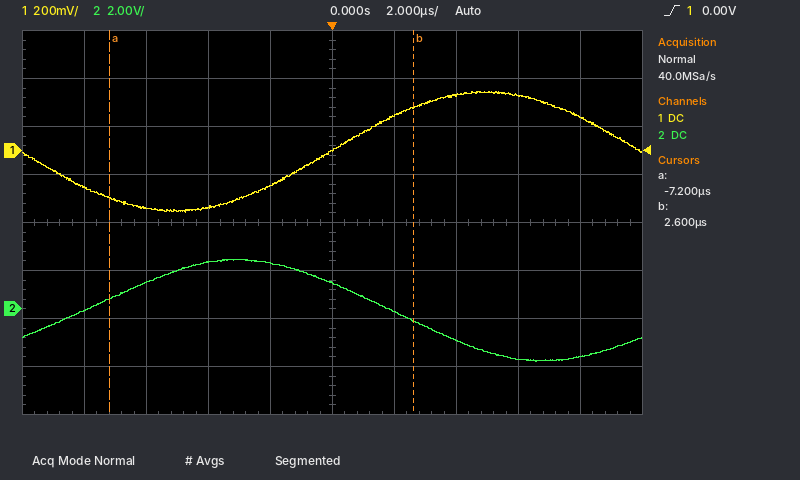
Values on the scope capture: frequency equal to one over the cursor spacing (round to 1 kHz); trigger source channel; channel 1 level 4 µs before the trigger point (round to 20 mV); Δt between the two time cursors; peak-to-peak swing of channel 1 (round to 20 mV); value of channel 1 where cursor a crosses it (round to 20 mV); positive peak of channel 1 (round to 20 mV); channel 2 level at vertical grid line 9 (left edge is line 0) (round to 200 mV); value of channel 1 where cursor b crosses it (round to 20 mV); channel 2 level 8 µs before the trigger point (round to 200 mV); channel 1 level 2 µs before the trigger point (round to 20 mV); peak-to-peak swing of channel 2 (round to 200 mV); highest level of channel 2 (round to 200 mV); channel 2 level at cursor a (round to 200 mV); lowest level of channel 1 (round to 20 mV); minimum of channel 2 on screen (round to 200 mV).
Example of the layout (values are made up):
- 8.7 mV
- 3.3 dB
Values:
- 102 kHz
- channel 1
- -240 mV
- 9.8 µs
- 500 mV
- -200 mV
- 240 mV
- -2.0 V
- 180 mV
- 0.0 V
- -140 mV
- 4.2 V
- 2.0 V
- 400 mV
- -260 mV
- -2.2 V
